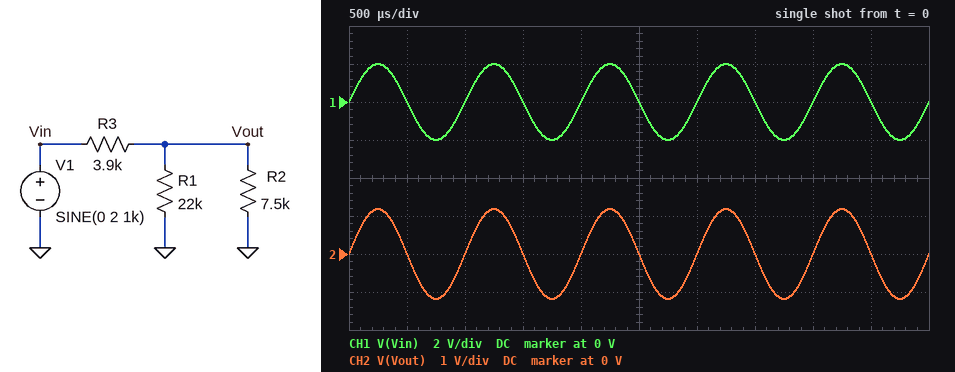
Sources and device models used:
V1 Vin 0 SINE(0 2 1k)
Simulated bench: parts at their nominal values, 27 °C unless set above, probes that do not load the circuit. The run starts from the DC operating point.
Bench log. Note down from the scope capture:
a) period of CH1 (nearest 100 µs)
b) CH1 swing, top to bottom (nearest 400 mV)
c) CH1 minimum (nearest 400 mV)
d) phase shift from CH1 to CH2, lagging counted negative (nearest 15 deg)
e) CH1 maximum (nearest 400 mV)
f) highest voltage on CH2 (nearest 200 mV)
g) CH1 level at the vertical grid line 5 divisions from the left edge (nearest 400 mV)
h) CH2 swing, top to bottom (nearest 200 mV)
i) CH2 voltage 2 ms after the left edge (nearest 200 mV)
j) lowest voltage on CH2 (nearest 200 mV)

1.0 ms
4.0 V
-2.0 V
0 deg
2.0 V
1.2 V
0 V
2.4 V
0 V
-1.2 V
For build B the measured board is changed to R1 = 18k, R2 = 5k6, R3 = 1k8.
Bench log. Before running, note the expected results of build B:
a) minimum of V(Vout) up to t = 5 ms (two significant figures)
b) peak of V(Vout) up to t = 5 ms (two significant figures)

-1.4 V
1.4 V
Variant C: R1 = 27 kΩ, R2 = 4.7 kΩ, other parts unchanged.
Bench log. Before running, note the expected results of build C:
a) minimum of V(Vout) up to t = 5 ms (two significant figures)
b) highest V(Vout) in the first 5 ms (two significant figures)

-1.0 V
1.0 V
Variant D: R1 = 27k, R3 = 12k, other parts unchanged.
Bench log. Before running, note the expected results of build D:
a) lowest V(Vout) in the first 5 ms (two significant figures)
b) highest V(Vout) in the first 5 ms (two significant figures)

-660 mV
660 mV
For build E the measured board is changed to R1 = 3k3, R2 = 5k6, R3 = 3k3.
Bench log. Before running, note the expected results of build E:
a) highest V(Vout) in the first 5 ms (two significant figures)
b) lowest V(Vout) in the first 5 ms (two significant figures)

770 mV
-770 mV
